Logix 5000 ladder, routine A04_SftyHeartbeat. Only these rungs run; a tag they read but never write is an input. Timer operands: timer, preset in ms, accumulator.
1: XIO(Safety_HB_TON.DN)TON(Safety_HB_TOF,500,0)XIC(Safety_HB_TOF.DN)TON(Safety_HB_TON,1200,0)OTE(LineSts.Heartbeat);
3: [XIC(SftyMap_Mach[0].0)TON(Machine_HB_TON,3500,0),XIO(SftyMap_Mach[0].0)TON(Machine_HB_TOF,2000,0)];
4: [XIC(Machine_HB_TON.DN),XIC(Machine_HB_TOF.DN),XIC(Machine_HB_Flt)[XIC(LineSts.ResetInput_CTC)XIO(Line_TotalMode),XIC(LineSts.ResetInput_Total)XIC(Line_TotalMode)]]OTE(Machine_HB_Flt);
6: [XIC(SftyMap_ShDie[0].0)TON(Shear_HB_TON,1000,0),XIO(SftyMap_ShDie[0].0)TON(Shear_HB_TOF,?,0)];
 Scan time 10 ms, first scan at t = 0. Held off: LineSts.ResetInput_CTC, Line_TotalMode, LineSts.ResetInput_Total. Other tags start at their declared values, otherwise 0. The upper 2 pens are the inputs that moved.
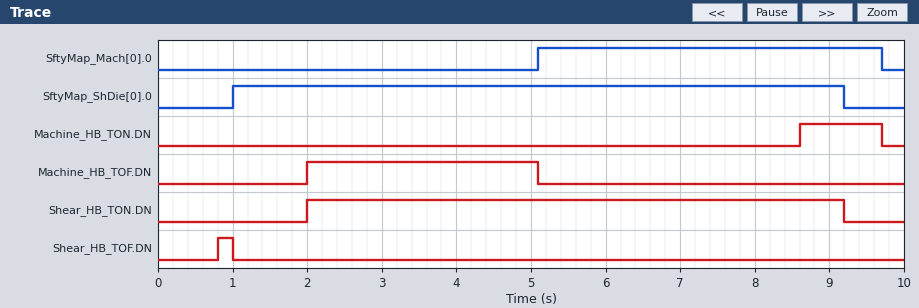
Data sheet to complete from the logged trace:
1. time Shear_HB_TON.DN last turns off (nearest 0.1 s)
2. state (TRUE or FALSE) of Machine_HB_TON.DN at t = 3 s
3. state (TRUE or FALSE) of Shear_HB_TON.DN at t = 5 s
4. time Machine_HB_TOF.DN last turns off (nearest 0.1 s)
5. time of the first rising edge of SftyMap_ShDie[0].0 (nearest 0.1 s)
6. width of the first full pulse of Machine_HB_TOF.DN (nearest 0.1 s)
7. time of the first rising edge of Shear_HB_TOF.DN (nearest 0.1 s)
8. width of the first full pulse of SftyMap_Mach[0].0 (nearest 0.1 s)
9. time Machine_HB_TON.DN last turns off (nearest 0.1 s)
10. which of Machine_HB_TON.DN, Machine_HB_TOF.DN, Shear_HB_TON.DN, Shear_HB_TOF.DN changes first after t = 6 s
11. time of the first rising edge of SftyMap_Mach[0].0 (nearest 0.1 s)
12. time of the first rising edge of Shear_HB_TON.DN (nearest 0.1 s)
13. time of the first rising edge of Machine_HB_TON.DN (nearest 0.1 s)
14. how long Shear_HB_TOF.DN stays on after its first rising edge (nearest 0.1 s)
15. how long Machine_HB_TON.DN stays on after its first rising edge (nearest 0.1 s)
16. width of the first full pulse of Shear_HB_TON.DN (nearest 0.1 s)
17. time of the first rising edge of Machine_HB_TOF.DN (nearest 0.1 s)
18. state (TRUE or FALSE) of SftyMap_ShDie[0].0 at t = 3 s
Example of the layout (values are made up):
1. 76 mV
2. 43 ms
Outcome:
1. 9.2 s
2. FALSE
3. TRUE
4. 5.1 s
5. 1.0 s
6. 3.1 s
7. 0.8 s
8. 4.6 s
9. 9.7 s
10. Machine_HB_TON.DN
11. 5.1 s
12. 2.0 s
13. 8.6 s
14. 0.2 s
15. 1.1 s
16. 7.2 s
17. 2.0 s
18. TRUE
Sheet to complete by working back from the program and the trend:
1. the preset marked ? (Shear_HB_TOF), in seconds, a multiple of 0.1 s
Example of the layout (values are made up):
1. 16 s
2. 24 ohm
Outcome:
1. 0.8 s
